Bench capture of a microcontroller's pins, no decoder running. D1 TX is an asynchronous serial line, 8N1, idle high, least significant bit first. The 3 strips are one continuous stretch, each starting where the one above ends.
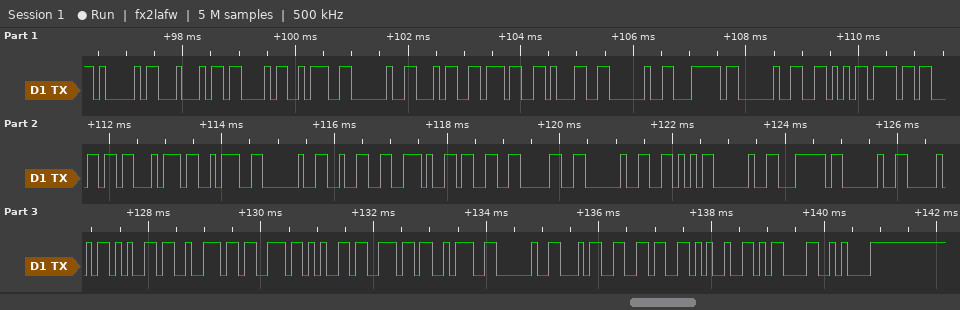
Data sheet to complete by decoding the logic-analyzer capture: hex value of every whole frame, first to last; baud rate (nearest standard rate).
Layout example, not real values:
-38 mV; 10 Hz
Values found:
41 44 43 3A 20 34 37 31 20 7C 20 56 6F 6C 74 3A 20 32 2E 33 30 20 56 20 7C 20 50 65 72 73 65 6E 3A 20 34 36 25 0D 0A; 9600 baud
